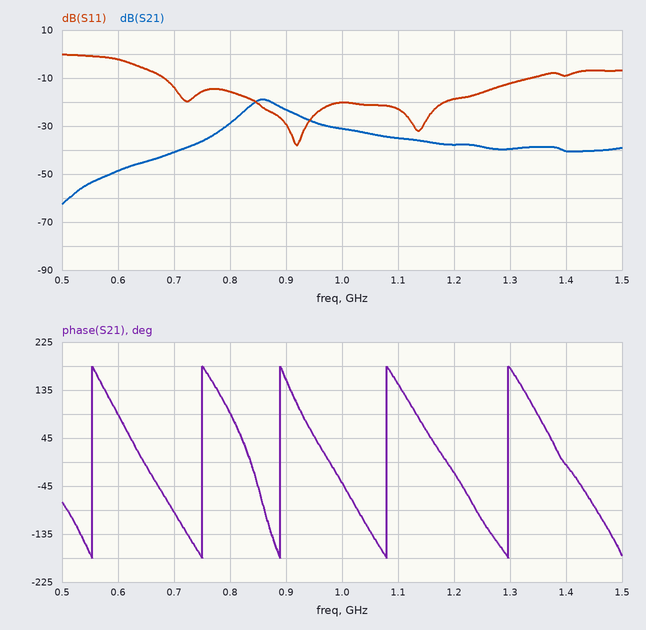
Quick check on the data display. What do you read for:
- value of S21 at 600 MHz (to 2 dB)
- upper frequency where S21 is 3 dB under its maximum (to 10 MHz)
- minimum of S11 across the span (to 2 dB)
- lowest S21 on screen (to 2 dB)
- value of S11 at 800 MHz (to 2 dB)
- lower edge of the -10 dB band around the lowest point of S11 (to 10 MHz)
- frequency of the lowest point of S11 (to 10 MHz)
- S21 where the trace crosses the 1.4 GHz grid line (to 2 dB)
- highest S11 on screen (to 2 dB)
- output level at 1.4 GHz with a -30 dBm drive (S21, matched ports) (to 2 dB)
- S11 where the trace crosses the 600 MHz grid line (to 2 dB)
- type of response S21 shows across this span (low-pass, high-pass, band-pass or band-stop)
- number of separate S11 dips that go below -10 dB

-48 dB
890 MHz
-38 dB
-62 dB
-16 dB
680 MHz
920 MHz
-40 dB
0 dB
-70 dBm
-2 dB
band-pass
3
